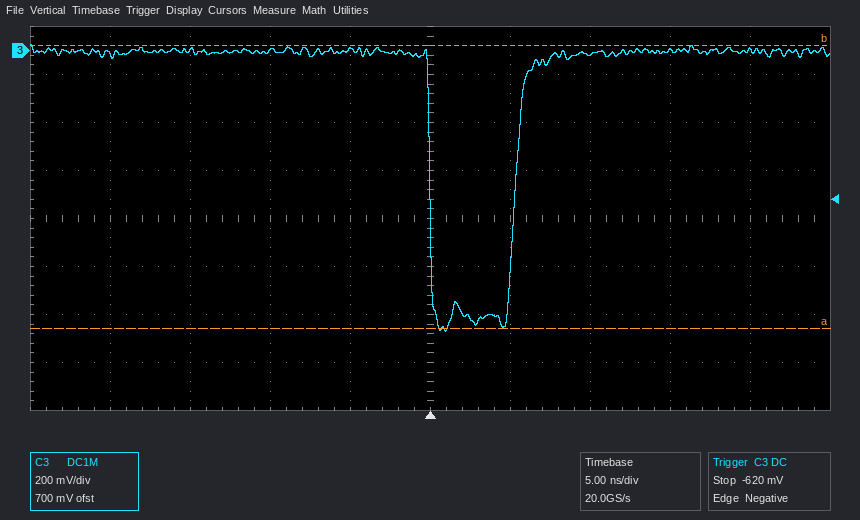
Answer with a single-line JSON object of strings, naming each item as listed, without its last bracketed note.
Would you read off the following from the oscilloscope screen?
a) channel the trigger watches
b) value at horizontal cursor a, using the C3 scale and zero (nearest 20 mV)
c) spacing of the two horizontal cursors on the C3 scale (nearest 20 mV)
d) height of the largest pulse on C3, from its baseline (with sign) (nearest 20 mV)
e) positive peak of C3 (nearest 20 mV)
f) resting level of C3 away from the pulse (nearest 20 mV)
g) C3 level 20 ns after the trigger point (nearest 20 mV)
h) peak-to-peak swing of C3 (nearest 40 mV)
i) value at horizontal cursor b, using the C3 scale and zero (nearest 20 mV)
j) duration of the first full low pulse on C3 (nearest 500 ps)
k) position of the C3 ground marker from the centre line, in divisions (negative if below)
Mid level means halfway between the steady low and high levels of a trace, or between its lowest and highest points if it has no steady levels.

{"channel the trigger watches": "C3", "value at horizontal cursor a, using the C3 scale and zero": "-1.16 V", "spacing of the two horizontal cursors on the C3 scale": "1.18 V", "height of the largest pulse on C3, from its baseline (with sign)": "-1.16 V", "positive peak of C3": "20 mV", "resting level of C3 away from the pulse": "0 mV", "C3 level 20 ns after the trigger point": "0 mV", "peak-to-peak swing of C3": "1.20 V", "value at horizontal cursor b, using the C3 scale and zero": "20 mV", "duration of the first full low pulse on C3": "5.5 ns", "position of the C3 ground marker from the centre line, in divisions": "+3.5 div"}
